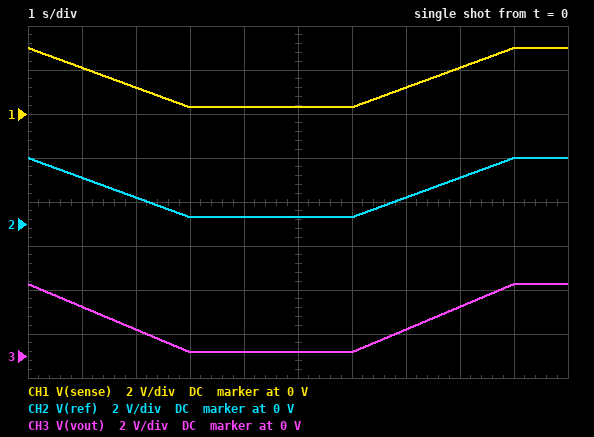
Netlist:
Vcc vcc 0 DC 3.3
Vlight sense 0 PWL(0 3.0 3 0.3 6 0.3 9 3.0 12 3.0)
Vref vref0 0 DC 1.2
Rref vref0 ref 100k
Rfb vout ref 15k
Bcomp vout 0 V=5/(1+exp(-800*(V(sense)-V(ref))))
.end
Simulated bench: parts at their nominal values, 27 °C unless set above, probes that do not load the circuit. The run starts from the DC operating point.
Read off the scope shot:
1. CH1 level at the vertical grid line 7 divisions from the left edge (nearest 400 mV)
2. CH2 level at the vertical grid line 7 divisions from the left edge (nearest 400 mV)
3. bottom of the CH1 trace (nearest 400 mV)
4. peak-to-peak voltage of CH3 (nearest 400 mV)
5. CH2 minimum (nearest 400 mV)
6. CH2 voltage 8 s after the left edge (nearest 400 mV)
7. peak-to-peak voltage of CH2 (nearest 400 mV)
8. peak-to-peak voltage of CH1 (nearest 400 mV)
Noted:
1.2 V
1.2 V
400 mV
3.2 V
400 mV
2.0 V
2.8 V
2.8 V
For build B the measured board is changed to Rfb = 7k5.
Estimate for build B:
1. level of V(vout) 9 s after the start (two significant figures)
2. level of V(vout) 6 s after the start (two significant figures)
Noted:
3.1 V
240 mV
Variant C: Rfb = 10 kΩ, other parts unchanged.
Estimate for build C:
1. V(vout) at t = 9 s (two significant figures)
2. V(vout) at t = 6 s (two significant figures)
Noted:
3.2 V
210 mV
